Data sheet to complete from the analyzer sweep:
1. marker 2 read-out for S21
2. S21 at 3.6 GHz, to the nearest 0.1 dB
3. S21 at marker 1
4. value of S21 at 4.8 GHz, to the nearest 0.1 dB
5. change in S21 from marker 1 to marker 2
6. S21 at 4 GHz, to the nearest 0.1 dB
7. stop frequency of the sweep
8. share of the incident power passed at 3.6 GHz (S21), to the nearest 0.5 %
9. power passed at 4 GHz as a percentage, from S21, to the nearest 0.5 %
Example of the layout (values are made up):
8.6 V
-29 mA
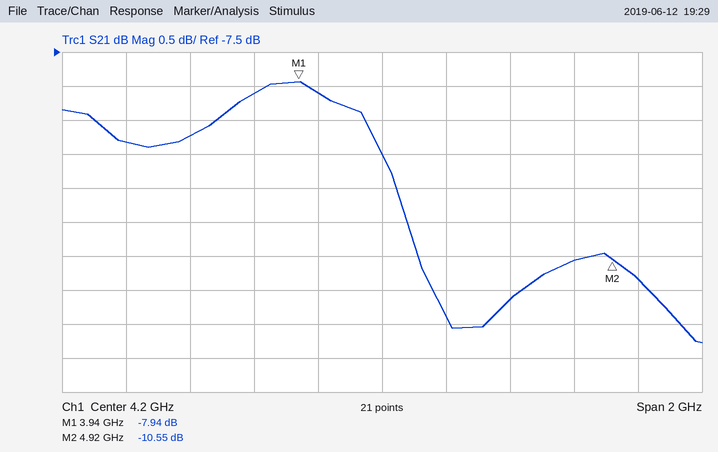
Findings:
-10.55 dB
-8.7 dB
-7.94 dB
-10.6 dB
-2.61 dB
-8.1 dB
5.2 GHz
13.5 %
15.5 %
